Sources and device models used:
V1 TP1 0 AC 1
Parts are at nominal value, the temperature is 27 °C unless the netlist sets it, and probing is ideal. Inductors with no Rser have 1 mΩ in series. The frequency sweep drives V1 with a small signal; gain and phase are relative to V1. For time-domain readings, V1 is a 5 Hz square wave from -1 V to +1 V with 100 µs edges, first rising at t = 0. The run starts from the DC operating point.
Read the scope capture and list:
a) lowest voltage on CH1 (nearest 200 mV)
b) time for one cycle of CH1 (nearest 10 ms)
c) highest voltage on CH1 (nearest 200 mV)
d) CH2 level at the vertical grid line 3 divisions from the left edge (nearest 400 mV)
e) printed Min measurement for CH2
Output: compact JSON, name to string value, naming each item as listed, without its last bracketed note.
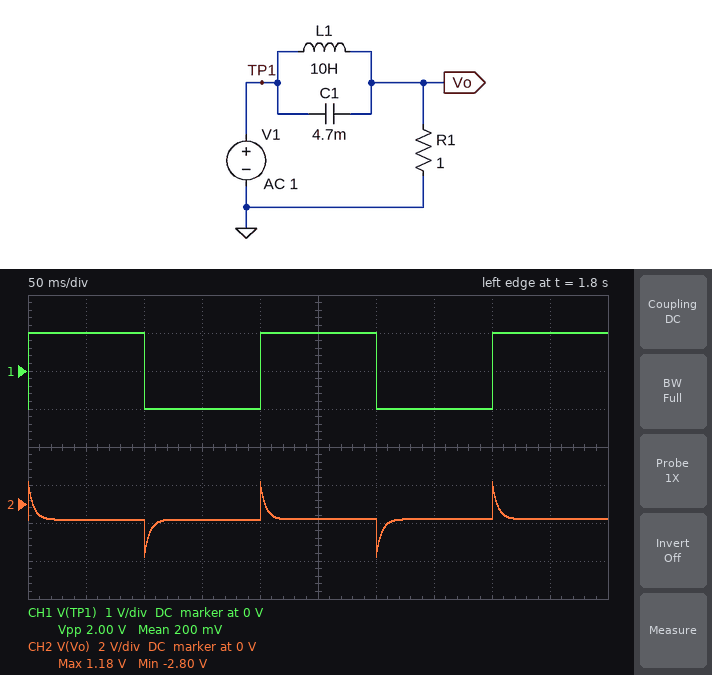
{"lowest voltage on CH1": "-1.0 V", "time for one cycle of CH1": "200 ms", "highest voltage on CH1": "1.0 V", "CH2 level at the vertical grid line 3 divisions from the left edge": "-800 mV", "printed Min measurement for CH2": "-2.80 V"}
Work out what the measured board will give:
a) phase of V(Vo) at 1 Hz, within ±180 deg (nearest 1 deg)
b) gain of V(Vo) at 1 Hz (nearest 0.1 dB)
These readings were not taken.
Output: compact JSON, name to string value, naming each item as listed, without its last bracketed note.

{"phase of V(Vo) at 1 Hz, within ±180 deg": "89 deg", "gain of V(Vo) at 1 Hz": "-37.3 dB"}
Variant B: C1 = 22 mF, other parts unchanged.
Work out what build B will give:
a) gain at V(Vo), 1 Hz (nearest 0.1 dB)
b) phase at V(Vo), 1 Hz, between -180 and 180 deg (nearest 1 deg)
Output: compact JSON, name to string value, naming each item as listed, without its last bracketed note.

{"gain at V(Vo), 1 Hz": "-18.3 dB", "phase at V(Vo), 1 Hz, between -180 and 180 deg": "83 deg"}
